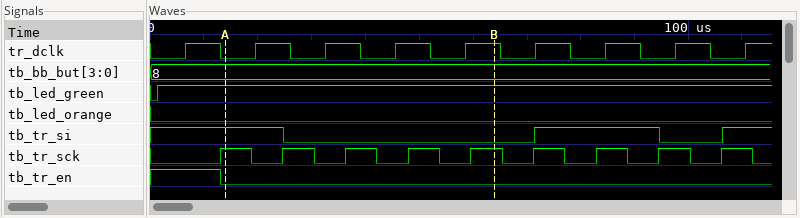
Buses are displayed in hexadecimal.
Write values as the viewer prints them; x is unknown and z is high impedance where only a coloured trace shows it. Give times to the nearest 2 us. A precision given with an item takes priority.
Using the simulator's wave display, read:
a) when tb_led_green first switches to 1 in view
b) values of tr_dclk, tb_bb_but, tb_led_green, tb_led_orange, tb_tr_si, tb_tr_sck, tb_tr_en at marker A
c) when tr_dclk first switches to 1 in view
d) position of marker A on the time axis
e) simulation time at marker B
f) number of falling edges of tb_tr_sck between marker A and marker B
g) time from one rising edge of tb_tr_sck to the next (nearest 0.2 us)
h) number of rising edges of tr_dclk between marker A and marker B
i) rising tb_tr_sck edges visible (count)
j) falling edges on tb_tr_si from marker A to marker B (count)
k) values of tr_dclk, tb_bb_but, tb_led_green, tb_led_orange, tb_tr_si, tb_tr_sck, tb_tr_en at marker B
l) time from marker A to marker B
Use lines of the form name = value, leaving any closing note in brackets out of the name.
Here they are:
when tb_led_green first switches to 1 in view = 2 us
values of tr_dclk, tb_bb_but, tb_led_green, tb_led_orange, tb_tr_si, tb_tr_sck, tb_tr_en at marker A = tr_dclk=0, tb_bb_but=8, tb_led_green=1, tb_led_orange=0, tb_tr_si=1, tb_tr_sck=1, tb_tr_en=0
when tr_dclk first switches to 1 in view = 6 us
position of marker A on the time axis = 14 us
simulation time at marker B = 64 us
number of falling edges of tb_tr_sck between marker A and marker B = 4
time from one rising edge of tb_tr_sck to the next = 11.6 us
number of rising edges of tr_dclk between marker A and marker B = 4
rising tb_tr_sck edges visible = 9
falling edges on tb_tr_si from marker A to marker B = 1
values of tr_dclk, tb_bb_but, tb_led_green, tb_led_orange, tb_tr_si, tb_tr_sck, tb_tr_en at marker B = tr_dclk=1, tb_bb_but=8, tb_led_green=1, tb_led_orange=0, tb_tr_si=0, tb_tr_sck=1, tb_tr_en=0
time from marker A to marker B = 50 us
